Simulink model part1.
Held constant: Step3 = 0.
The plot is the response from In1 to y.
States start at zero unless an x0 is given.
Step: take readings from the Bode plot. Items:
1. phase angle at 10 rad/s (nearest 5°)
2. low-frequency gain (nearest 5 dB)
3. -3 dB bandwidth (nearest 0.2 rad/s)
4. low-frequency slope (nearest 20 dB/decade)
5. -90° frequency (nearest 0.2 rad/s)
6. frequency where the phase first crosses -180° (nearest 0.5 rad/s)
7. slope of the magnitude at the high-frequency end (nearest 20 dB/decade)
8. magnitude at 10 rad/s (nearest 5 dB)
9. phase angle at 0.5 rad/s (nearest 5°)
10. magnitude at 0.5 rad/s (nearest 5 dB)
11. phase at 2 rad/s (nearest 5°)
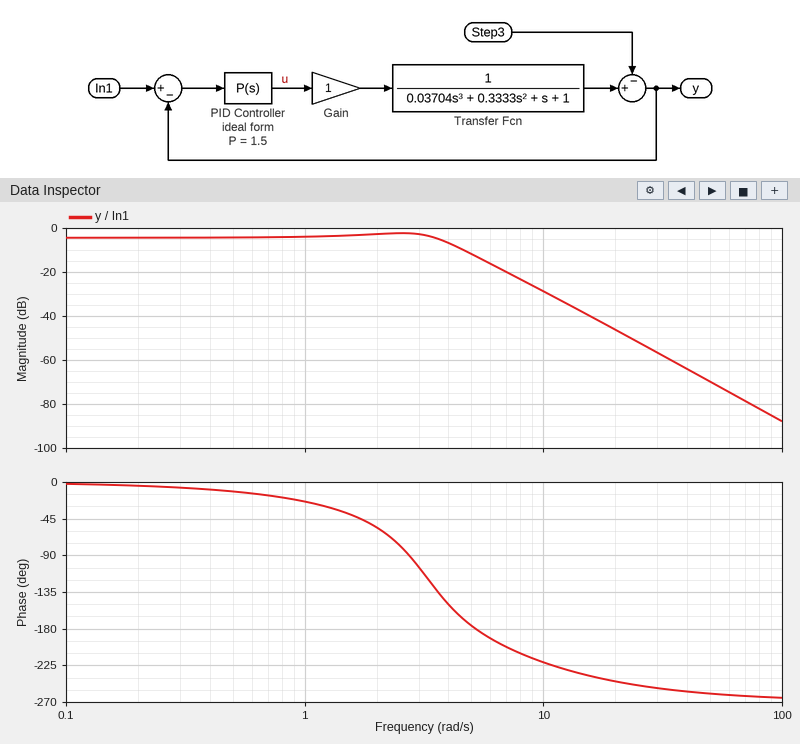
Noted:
-220°
-5 dB
4.2 rad/s
0 dB/decade
2.8 rad/s
5.0 rad/s
-60 dB/decade
-30 dB
-10°
-5 dB
-55°
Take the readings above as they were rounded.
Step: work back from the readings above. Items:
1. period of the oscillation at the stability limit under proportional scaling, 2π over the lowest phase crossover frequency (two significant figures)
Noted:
1.3 s
